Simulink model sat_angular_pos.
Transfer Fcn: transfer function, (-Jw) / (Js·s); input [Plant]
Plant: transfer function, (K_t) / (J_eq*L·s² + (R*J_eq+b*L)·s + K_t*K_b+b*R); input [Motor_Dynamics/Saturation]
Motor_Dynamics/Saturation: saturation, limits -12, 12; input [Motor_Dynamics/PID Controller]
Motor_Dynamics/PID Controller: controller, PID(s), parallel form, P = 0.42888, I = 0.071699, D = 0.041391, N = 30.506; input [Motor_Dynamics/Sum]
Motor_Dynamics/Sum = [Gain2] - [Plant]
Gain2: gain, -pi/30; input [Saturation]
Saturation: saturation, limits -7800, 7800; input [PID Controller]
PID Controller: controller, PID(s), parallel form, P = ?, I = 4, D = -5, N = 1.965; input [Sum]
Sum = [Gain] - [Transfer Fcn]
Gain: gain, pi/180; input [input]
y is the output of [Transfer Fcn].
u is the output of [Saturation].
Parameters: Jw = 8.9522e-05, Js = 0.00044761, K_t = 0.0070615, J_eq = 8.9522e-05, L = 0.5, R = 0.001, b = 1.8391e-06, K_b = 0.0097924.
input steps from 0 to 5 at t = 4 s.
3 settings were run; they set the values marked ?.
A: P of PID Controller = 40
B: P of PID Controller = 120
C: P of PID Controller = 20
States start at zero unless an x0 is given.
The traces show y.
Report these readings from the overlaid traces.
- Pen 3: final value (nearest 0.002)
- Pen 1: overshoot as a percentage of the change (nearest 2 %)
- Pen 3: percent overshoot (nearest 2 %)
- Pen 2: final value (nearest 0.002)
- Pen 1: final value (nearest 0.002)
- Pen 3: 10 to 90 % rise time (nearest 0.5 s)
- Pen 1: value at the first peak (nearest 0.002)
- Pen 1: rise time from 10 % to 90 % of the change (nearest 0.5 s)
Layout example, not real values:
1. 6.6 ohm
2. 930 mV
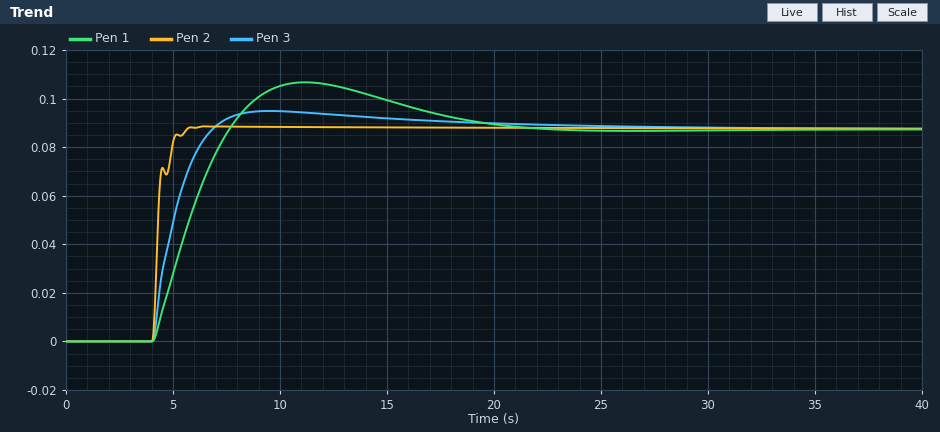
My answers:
1. 0.088
2. 22 %
3. 8 %
4. 0.088
5. 0.088
6. 2.0 s
7. 0.106
8. 2.5 s
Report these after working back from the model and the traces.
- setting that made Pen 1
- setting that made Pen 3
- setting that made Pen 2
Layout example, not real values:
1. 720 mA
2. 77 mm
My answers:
1. C
2. A
3. B
